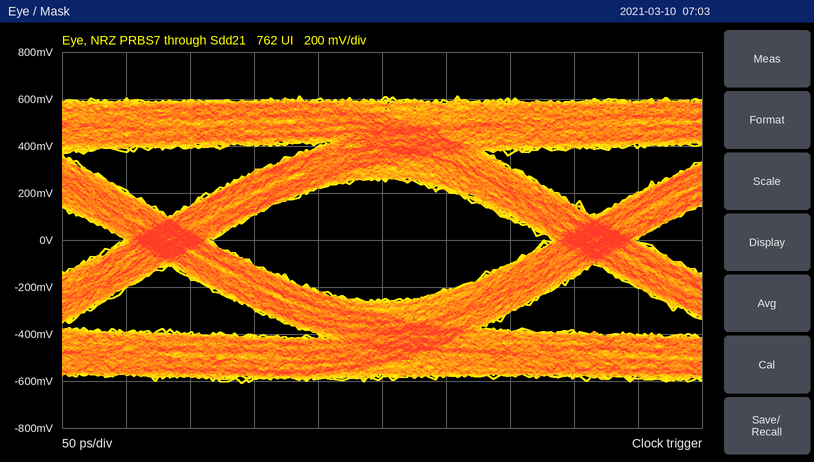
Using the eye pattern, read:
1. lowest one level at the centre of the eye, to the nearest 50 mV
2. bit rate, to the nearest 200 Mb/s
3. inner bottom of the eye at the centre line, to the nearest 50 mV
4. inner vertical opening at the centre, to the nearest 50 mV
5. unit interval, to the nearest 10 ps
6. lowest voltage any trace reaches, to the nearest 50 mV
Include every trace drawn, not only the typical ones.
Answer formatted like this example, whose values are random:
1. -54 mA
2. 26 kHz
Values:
1. 250 mV
2. 3.0 Gb/s
3. -250 mV
4. 500 mV
5. 330 ps
6. -600 mV
